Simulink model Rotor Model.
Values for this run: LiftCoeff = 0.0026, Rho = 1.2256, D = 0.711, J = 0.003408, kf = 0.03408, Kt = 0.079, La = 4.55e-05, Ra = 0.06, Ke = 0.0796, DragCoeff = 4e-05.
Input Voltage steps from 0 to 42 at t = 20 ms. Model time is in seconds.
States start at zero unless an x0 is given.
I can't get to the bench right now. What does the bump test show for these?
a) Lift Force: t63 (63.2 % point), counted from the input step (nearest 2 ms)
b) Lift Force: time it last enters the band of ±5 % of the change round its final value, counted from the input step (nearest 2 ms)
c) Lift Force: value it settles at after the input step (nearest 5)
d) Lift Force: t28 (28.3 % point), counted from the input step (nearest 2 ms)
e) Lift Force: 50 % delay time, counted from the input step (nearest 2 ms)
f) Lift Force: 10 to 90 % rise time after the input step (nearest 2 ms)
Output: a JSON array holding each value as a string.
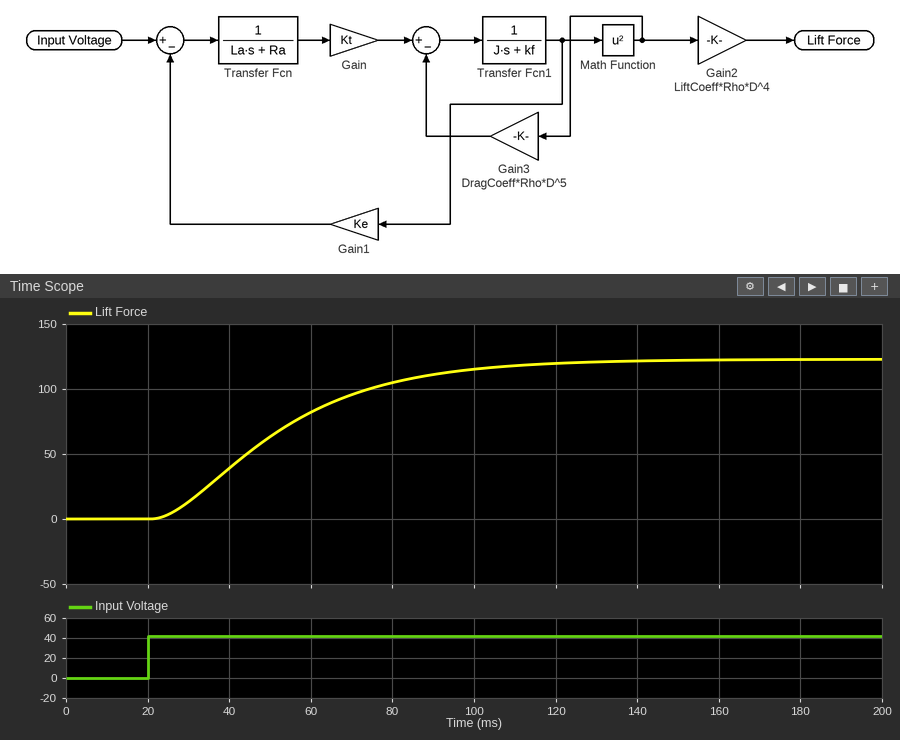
["38 ms", "86 ms", "125", "18 ms", "30 ms", "60 ms"]
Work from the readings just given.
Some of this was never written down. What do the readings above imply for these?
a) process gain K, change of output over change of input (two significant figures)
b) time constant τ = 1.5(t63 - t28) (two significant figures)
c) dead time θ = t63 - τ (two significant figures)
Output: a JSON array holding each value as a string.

["3.0", "30 ms", "8.0 ms"]
